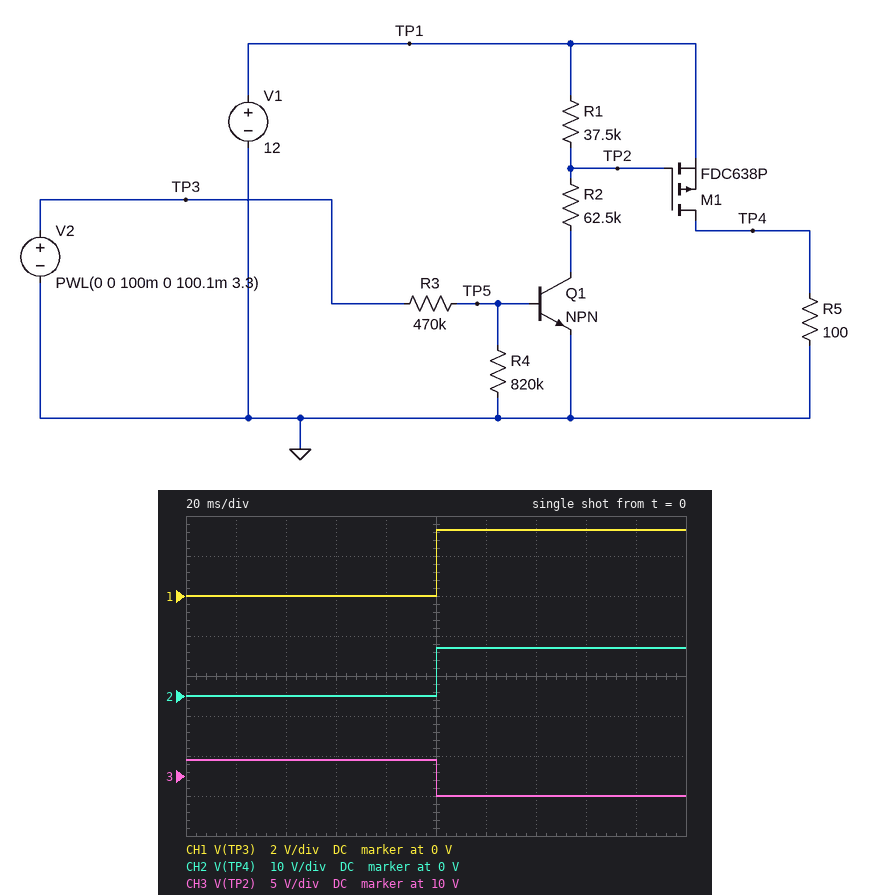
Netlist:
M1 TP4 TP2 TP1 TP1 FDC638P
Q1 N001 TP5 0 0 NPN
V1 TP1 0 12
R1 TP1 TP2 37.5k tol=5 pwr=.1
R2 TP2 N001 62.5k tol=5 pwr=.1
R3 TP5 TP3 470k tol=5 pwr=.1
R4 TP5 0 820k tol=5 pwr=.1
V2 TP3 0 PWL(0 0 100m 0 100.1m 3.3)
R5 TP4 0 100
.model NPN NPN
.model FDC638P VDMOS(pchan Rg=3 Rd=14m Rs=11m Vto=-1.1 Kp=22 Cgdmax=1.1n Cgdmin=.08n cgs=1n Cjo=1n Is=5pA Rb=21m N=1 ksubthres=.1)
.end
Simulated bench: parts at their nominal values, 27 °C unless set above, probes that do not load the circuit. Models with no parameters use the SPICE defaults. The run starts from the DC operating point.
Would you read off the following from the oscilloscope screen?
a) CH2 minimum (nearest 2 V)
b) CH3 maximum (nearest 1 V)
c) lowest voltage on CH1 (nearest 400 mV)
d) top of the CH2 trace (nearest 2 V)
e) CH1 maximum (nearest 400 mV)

0 V
12 V
0 V
12 V
3.2 V
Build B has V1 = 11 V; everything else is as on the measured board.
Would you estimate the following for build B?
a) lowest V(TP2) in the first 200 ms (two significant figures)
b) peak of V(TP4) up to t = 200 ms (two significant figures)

6.9 V
11 V
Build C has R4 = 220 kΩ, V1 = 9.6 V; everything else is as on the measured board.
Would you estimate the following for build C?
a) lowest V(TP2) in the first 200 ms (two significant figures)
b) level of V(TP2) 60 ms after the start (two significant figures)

6.0 V
9.6 V
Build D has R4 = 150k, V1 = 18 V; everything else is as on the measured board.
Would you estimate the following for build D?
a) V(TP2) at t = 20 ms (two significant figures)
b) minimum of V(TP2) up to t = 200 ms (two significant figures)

18 V
15 V
